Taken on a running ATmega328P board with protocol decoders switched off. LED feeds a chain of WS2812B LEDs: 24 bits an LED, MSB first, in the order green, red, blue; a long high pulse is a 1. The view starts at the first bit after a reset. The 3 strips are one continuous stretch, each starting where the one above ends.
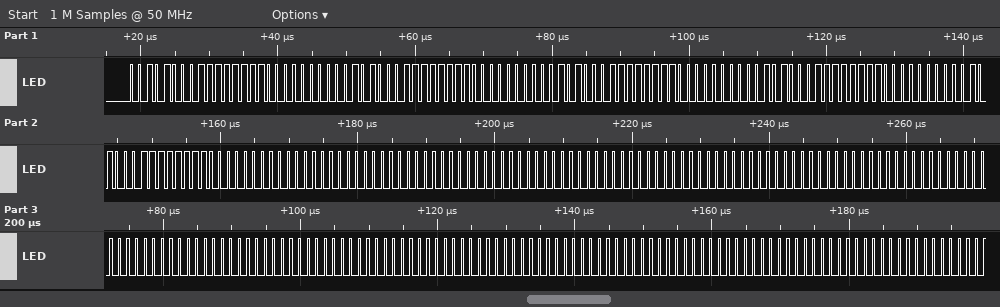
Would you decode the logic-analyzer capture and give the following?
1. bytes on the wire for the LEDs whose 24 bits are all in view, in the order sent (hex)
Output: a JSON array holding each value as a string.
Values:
["28 FF 00 28 FF 00 28 FF 00 28 FF 00 28 FF 00 00 00 00 00 00 00 00 00 00 00 00 00 00 00 00 00 00 00 00 00 00"]
